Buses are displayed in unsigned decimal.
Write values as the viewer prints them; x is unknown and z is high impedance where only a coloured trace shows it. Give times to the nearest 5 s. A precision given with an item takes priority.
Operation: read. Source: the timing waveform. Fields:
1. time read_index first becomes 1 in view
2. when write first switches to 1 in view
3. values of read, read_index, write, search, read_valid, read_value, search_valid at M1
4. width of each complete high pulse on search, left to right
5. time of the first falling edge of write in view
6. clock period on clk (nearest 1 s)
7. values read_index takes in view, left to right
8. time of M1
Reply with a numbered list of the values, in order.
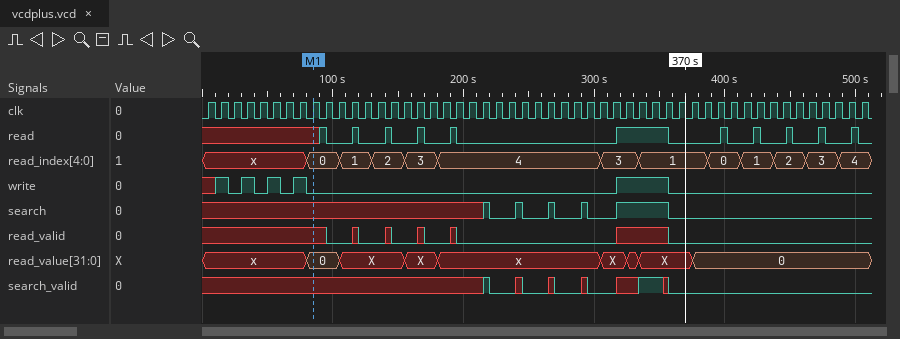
1. 105 s
2. 10 s
3. read=x, read_index=0, write=0, search=x, read_valid=x, read_value=0, search_valid=x
4. 5 s, 5 s, 5 s, 40 s
5. 20 s
6. 10 s
7. x, 0, 1, 2, 3, 4, 3, 1, 0, 1, 2, 3, 4
8. 85 s
